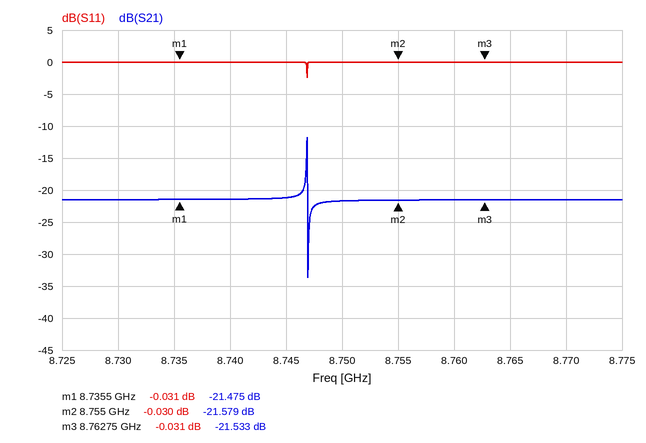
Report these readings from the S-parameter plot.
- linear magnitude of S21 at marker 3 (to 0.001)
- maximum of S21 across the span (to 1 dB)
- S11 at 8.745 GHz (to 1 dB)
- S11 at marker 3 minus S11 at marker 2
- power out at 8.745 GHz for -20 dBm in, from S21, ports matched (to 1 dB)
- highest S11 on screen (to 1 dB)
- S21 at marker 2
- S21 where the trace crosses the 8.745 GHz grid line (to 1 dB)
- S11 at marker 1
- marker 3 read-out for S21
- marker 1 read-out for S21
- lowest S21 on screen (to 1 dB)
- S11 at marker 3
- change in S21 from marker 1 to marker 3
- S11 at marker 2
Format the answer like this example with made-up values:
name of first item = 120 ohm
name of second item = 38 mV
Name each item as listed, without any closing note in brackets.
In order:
linear magnitude of S21 at marker 3 = 0.084
maximum of S21 across the span = -12 dB
S11 at 8.745 GHz = 0 dB
S11 at marker 3 minus S11 at marker 2 = -0.001 dB
power out at 8.745 GHz for -20 dBm in, from S21, ports matched = -41 dBm
highest S11 on screen = 0 dB
S21 at marker 2 = -21.579 dB
S21 where the trace crosses the 8.745 GHz grid line = -21 dB
S11 at marker 1 = -0.031 dB
marker 3 read-out for S21 = -21.533 dB
marker 1 read-out for S21 = -21.475 dB
lowest S21 on screen = -34 dB
S11 at marker 3 = -0.031 dB
change in S21 from marker 1 to marker 3 = -0.058 dB
S11 at marker 2 = -0.030 dB
